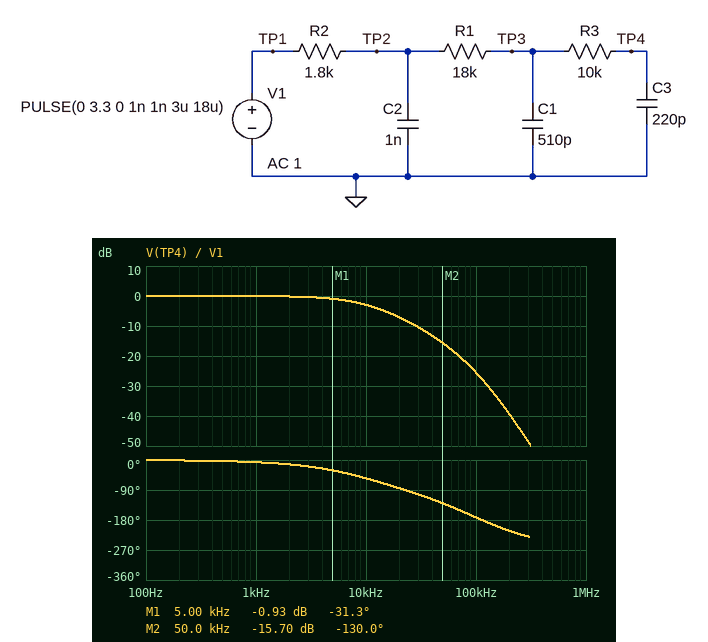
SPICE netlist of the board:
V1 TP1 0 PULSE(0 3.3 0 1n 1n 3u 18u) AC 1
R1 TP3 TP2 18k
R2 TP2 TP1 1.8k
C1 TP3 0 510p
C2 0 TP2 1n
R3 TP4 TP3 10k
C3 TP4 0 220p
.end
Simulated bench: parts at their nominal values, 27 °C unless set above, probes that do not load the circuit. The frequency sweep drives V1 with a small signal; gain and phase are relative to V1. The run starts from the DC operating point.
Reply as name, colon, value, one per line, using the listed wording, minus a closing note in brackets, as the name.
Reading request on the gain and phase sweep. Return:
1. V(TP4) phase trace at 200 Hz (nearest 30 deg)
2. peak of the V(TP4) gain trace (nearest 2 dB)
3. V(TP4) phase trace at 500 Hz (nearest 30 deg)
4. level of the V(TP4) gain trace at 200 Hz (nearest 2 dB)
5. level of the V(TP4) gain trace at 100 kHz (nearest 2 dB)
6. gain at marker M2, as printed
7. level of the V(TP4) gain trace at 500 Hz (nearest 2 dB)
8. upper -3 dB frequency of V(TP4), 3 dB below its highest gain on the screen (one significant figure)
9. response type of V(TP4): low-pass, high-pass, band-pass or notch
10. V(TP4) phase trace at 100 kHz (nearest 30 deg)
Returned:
V(TP4) phase trace at 200 Hz: 0 deg
peak of the V(TP4) gain trace: 0 dB
V(TP4) phase trace at 500 Hz: 0 deg
level of the V(TP4) gain trace at 200 Hz: 0 dB
level of the V(TP4) gain trace at 100 kHz: -26 dB
gain at marker M2, as printed: -15.70 dB
level of the V(TP4) gain trace at 500 Hz: 0 dB
upper -3 dB frequency of V(TP4), 3 dB below its highest gain on the screen: 10 kHz
response type of V(TP4): low-pass, high-pass, band-pass or notch: low-pass
V(TP4) phase trace at 100 kHz: -180 deg
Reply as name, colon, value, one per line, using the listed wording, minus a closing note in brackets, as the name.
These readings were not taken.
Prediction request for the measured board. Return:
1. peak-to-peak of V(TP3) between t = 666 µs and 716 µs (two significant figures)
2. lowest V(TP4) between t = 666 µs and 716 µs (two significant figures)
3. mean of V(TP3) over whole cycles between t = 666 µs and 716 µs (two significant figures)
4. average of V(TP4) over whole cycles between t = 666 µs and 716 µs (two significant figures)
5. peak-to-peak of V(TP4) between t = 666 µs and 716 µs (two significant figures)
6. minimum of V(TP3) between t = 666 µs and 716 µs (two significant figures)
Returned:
peak-to-peak of V(TP3) between t = 666 µs and 716 µs: 450 mV
lowest V(TP4) between t = 666 µs and 716 µs: 380 mV
mean of V(TP3) over whole cycles between t = 666 µs and 716 µs: 550 mV
average of V(TP4) over whole cycles between t = 666 µs and 716 µs: 550 mV
peak-to-peak of V(TP4) between t = 666 µs and 716 µs: 320 mV
minimum of V(TP3) between t = 666 µs and 716 µs: 340 mV
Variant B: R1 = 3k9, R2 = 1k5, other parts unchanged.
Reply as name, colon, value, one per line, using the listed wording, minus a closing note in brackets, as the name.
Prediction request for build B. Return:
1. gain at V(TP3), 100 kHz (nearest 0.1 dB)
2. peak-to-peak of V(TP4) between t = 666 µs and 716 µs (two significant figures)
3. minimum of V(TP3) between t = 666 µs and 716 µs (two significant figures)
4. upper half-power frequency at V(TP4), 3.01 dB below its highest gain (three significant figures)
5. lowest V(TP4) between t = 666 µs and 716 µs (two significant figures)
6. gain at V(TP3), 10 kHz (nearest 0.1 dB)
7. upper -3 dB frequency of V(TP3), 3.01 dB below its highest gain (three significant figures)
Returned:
gain at V(TP3), 100 kHz: -10.0 dB
peak-to-peak of V(TP4) between t = 666 µs and 716 µs: 940 mV
minimum of V(TP3) between t = 666 µs and 716 µs: 85 mV
upper half-power frequency at V(TP4), 3.01 dB below its highest gain: 27.4 kHz
lowest V(TP4) between t = 666 µs and 716 µs: 140 mV
gain at V(TP3), 10 kHz: -0.4 dB
upper -3 dB frequency of V(TP3), 3.01 dB below its highest gain: 31.9 kHz
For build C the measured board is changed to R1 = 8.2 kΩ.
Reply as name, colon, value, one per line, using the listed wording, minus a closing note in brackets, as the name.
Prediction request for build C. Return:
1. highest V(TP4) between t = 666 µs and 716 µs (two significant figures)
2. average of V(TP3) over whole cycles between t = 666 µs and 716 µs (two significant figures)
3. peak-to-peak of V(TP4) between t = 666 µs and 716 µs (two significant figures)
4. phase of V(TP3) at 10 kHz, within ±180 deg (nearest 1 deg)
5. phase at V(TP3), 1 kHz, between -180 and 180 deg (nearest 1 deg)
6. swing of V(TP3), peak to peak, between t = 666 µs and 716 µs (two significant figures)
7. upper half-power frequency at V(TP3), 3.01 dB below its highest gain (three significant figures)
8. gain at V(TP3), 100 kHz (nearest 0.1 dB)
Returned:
highest V(TP4) between t = 666 µs and 716 µs: 850 mV
average of V(TP3) over whole cycles between t = 666 µs and 716 µs: 550 mV
peak-to-peak of V(TP4) between t = 666 µs and 716 µs: 590 mV
phase of V(TP3) at 10 kHz, within ±180 deg: -30 deg
phase at V(TP3), 1 kHz, between -180 and 180 deg: -3 deg
swing of V(TP3), peak to peak, between t = 666 µs and 716 µs: 830 mV
upper half-power frequency at V(TP3), 3.01 dB below its highest gain: 19.0 kHz
gain at V(TP3), 100 kHz: -15.1 dB
